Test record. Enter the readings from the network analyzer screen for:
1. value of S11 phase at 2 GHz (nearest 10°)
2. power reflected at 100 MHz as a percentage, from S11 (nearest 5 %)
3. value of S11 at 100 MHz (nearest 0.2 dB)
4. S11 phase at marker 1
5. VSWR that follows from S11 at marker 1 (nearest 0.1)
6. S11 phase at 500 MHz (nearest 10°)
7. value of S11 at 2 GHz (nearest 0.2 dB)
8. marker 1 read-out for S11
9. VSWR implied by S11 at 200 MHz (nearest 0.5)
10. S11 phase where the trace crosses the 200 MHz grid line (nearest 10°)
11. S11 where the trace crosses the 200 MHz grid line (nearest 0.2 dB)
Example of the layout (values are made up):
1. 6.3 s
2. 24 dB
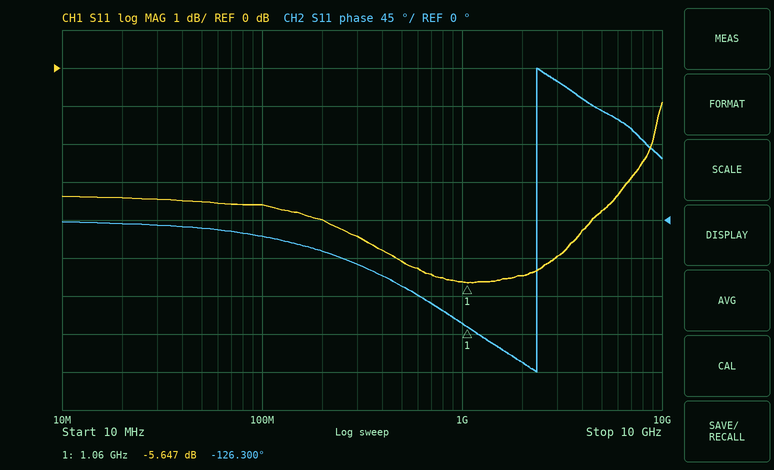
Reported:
1. -170°
2. 45 %
3. -3.6 dB
4. -126.300°
5. 3.2
6. -80°
7. -5.4 dB
8. -5.647 dB
9. 4.5
10. -40°
11. -4.0 dB
